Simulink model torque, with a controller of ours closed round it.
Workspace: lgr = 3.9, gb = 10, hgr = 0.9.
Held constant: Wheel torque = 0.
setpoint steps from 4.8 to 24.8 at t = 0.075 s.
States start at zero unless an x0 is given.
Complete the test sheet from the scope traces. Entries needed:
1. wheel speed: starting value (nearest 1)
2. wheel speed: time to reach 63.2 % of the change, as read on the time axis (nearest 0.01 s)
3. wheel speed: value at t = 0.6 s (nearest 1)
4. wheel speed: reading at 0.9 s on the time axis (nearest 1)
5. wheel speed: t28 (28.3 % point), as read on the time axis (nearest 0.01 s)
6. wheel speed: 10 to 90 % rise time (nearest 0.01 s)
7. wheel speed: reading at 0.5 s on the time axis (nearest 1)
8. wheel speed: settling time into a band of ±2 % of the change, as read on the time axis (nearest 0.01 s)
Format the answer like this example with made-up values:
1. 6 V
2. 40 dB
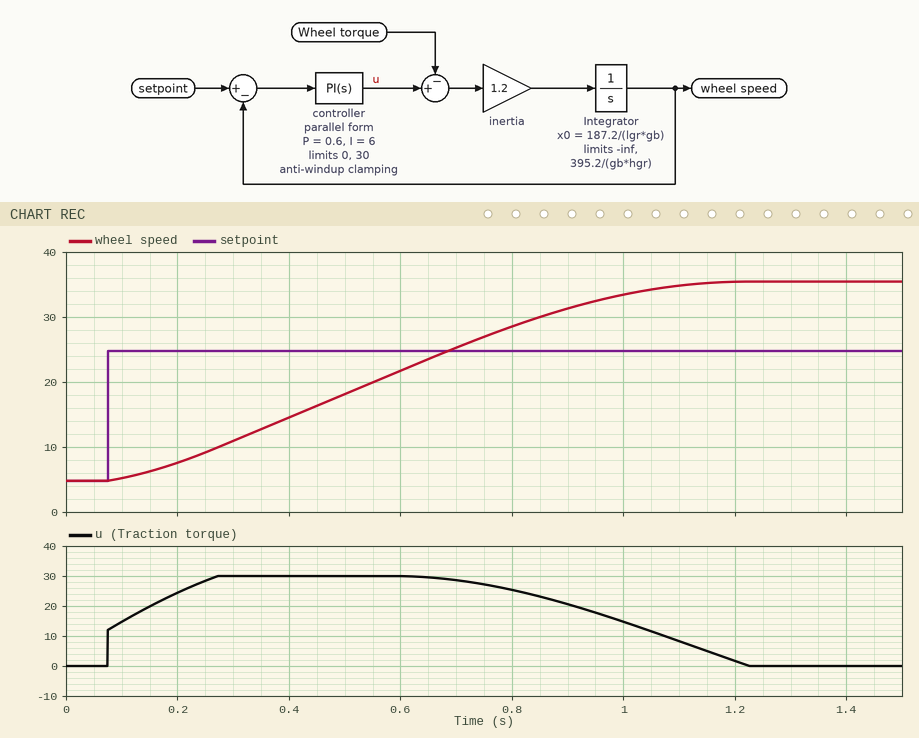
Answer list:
1. 5
2. 0.67 s
3. 22
4. 31
5. 0.37 s
6. 0.74 s
7. 18
8. 1.10 s
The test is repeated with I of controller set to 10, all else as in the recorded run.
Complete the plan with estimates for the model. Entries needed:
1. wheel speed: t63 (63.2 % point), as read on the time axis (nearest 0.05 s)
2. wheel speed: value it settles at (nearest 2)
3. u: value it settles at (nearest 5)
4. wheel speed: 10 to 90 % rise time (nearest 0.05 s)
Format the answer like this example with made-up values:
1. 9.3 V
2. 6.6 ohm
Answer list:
1. 0.60 s
2. 34
3. 0
4. 0.65 s
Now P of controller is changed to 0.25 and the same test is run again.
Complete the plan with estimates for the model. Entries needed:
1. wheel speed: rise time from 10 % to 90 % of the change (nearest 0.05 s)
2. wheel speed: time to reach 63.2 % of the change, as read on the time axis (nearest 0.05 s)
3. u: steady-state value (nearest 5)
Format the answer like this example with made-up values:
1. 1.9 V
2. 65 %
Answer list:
1. 0.75 s
2. 0.75 s
3. 0
